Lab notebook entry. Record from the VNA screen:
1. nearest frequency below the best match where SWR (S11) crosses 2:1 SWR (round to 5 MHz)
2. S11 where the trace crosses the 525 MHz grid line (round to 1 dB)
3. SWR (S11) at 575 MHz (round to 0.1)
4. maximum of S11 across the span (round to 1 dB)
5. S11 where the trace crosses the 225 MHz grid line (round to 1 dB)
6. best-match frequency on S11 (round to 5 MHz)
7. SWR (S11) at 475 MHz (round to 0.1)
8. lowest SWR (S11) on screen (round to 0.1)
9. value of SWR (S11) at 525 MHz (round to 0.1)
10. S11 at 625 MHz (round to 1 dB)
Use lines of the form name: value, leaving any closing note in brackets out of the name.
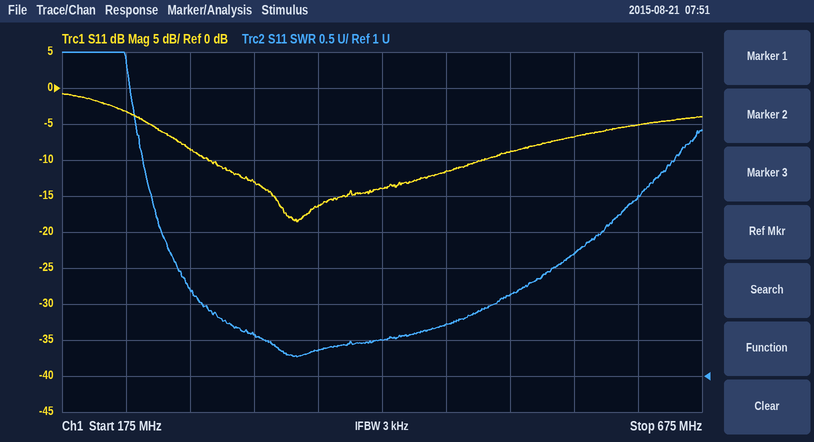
nearest frequency below the best match where SWR (S11) crosses 2:1 SWR: 285 MHz
S11 where the trace crosses the 525 MHz grid line: -9 dB
SWR (S11) at 575 MHz: 2.7
maximum of S11 across the span: -1 dB
S11 where the trace crosses the 225 MHz grid line: -3 dB
best-match frequency on S11: 360 MHz
SWR (S11) at 475 MHz: 1.7
lowest SWR (S11) on screen: 1.3
value of SWR (S11) at 525 MHz: 2.1
S11 at 625 MHz: -5 dB
